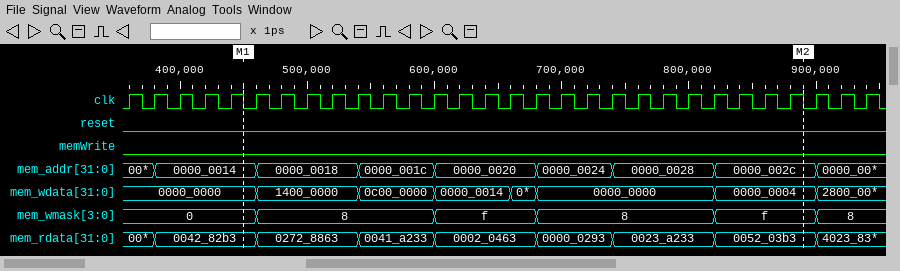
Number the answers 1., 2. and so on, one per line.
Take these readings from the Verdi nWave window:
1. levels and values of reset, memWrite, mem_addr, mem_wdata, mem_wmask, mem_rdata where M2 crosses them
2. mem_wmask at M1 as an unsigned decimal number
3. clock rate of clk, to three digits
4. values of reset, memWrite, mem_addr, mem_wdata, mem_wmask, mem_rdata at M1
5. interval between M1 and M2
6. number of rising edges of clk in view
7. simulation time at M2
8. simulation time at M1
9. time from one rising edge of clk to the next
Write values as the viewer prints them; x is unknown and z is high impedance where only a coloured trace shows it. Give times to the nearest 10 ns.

1. reset=0, memWrite=0, mem_addr=0000_002c, mem_wdata=0000_0004, mem_wmask=f, mem_rdata=0052_03b3
2. 0
3. 50.0 MHz
4. reset=0, memWrite=0, mem_addr=0000_0014, mem_wdata=0000_0000, mem_wmask=0, mem_rdata=0042_82b3
5. 440 ns
6. 30
7. 890 ns
8. 450 ns
9. 20 ns
